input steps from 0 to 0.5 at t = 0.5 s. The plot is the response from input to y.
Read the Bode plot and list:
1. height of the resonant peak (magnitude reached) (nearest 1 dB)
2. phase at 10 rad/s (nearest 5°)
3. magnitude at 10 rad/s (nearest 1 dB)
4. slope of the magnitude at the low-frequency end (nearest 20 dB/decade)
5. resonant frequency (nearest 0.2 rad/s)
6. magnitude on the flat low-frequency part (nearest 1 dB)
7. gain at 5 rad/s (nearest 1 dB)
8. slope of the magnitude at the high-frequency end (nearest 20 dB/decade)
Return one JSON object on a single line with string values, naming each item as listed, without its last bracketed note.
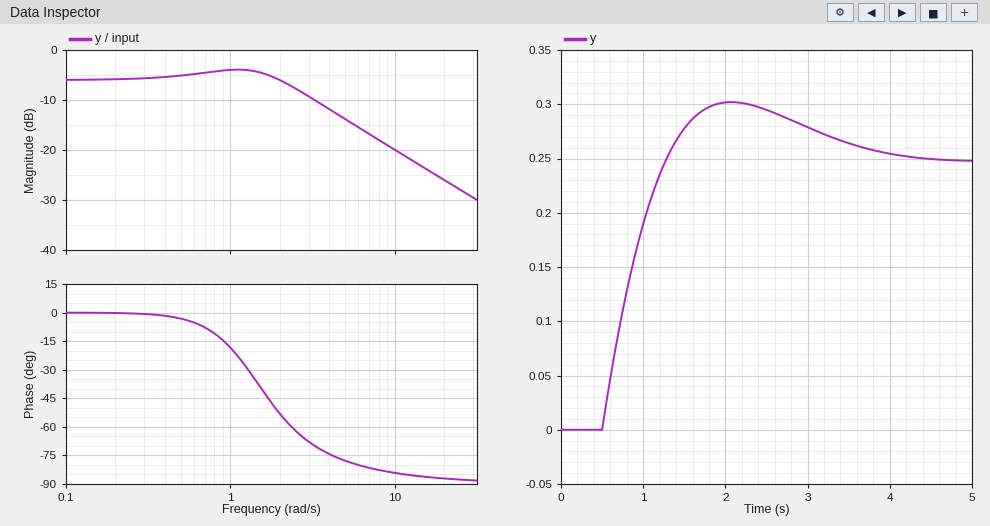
{"height of the resonant peak (magnitude reached)": "-4 dB", "phase at 10 rad/s": "-85°", "magnitude at 10 rad/s": "-20 dB", "slope of the magnitude at the low-frequency end": "0 dB/decade", "resonant frequency": "1.0 rad/s", "magnitude on the flat low-frequency part": "-6 dB", "gain at 5 rad/s": "-14 dB", "slope of the magnitude at the high-frequency end": "-20 dB/decade"}
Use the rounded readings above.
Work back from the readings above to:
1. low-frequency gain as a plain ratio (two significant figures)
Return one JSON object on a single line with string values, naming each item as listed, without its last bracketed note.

{"low-frequency gain as a plain ratio": "0.50"}
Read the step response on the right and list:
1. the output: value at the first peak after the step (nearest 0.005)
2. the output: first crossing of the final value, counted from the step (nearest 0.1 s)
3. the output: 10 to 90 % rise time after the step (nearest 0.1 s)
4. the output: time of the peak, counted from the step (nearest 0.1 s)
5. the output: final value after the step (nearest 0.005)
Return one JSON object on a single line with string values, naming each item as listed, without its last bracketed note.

{"the output: value at the first peak after the step": "0.300", "the output: first crossing of the final value, counted from the step": "0.8 s", "the output: 10 to 90 % rise time after the step": "0.6 s", "the output: time of the peak, counted from the step": "1.6 s", "the output: final value after the step": "0.250"}
